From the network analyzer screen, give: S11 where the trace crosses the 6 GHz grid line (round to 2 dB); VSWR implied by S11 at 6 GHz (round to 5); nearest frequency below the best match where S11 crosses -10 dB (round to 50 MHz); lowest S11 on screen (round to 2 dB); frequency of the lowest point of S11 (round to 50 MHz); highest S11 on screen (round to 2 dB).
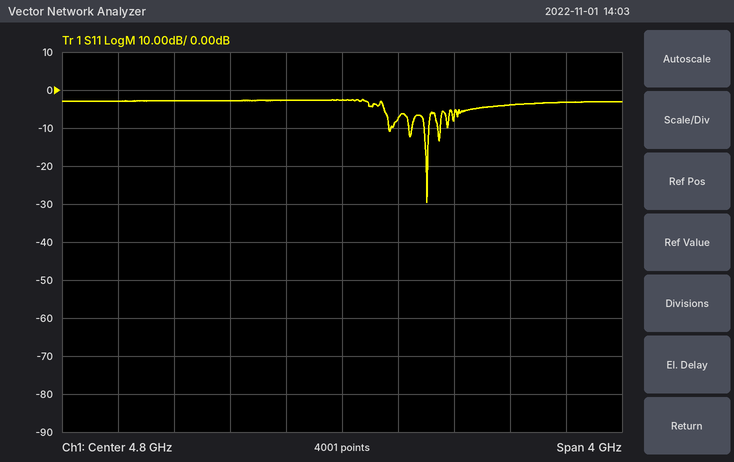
-4 dB
5
5.40 GHz
-30 dB
5.40 GHz
-2 dB
